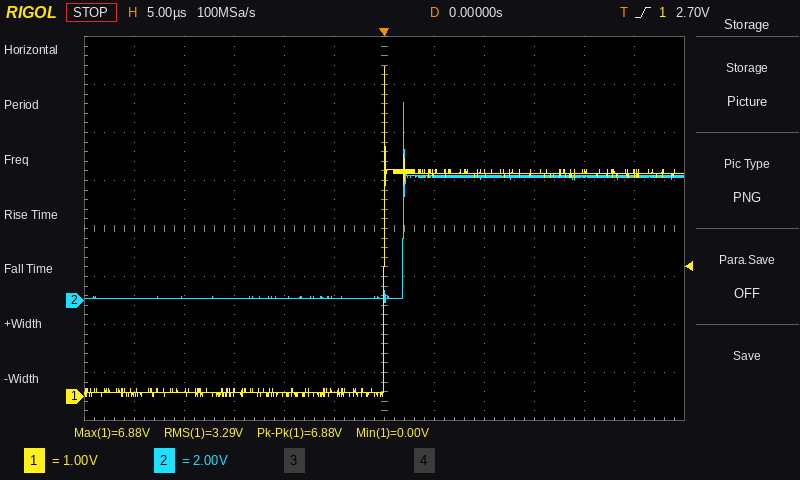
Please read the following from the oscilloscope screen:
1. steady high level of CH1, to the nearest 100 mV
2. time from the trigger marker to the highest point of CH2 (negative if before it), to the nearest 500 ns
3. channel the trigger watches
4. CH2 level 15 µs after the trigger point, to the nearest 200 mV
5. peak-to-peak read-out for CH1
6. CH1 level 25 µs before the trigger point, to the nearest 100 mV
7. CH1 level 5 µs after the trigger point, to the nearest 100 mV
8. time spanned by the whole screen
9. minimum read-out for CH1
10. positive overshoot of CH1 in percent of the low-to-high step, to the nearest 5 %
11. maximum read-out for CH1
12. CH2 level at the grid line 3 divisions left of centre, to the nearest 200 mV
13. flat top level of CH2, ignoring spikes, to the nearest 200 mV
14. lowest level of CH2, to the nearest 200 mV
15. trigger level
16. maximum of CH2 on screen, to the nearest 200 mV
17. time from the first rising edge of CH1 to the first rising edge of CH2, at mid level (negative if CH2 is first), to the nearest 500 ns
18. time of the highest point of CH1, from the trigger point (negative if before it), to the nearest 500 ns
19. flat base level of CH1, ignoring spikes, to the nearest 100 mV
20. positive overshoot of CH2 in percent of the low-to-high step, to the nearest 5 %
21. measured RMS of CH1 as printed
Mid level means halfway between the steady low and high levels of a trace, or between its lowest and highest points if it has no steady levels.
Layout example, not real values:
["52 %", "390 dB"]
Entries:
["4.6 V", "+2.0 µs", "CH1", "5.2 V", "6.88 V", "100 mV", "4.6 V", "60 µs", "0.00 V", "50 %", "6.88 V", "0.0 V", "5.2 V", "0.0 V", "2.70 V", "8.2 V", "+2.0 µs", "0.0 µs", "100 mV", "60 %", "3.29 V"]
